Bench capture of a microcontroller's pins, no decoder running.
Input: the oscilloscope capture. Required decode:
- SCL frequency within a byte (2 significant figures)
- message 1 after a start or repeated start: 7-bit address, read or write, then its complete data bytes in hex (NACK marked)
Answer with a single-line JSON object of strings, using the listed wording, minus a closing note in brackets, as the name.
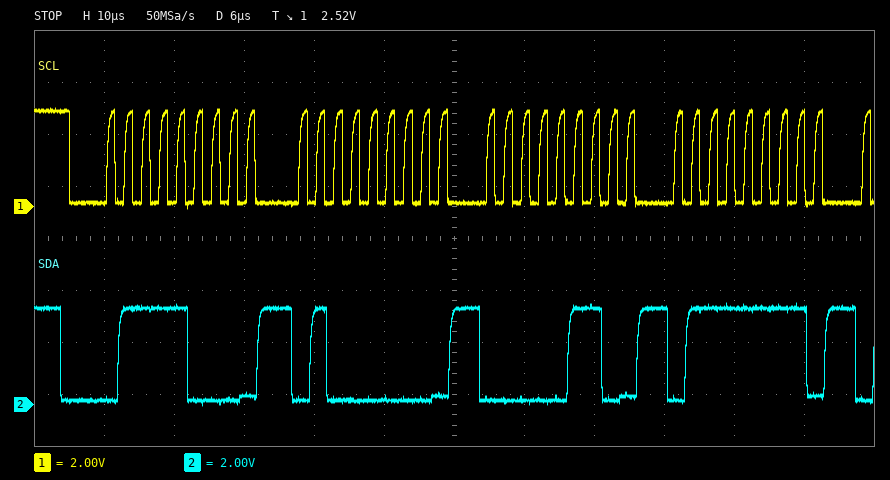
{"SCL frequency within a byte": "400 kHz", "message 1 after a start or repeated start: 7-bit address, read or write, then its complete data bytes in hex": "0x3C write: 40 06 7F"}
